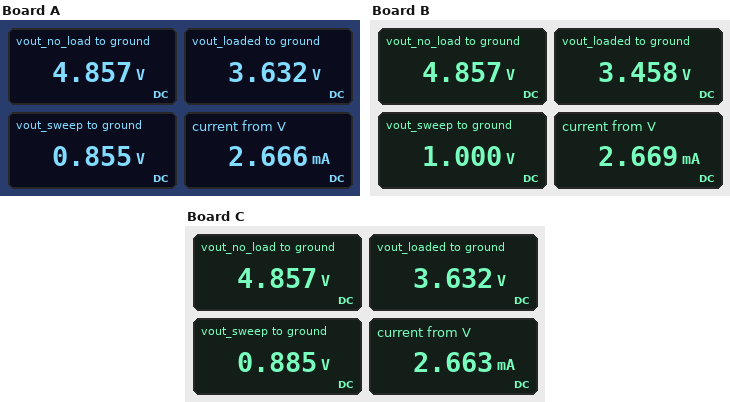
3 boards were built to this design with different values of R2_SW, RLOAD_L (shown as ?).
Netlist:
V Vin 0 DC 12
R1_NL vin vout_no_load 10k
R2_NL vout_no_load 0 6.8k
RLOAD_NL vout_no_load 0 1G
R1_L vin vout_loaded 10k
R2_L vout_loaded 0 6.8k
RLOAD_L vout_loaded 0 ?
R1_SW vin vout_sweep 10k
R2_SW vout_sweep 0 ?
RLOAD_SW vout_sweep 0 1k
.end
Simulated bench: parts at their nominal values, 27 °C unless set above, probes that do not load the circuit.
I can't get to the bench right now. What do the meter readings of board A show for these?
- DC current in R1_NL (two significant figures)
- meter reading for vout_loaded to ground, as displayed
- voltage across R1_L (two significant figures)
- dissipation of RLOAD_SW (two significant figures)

710 µA
3.632 V
8.4 V
730 µW
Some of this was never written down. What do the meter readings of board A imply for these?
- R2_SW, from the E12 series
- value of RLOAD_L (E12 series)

3.3 kΩ
12 kΩ
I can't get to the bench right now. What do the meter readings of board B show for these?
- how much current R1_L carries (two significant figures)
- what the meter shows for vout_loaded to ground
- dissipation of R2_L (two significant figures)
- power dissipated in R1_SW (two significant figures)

850 µA
3.458 V
1.8 mW
12 mW
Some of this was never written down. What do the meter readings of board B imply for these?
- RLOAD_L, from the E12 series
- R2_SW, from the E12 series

10 kΩ
10 kΩ
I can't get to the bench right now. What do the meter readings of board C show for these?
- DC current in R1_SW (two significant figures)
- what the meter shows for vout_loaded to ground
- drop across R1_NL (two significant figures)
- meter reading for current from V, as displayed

1.1 mA
3.632 V
7.1 V
2.663 mA
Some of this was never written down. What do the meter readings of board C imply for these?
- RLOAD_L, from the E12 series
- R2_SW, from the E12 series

12 kΩ
3.9 kΩ
